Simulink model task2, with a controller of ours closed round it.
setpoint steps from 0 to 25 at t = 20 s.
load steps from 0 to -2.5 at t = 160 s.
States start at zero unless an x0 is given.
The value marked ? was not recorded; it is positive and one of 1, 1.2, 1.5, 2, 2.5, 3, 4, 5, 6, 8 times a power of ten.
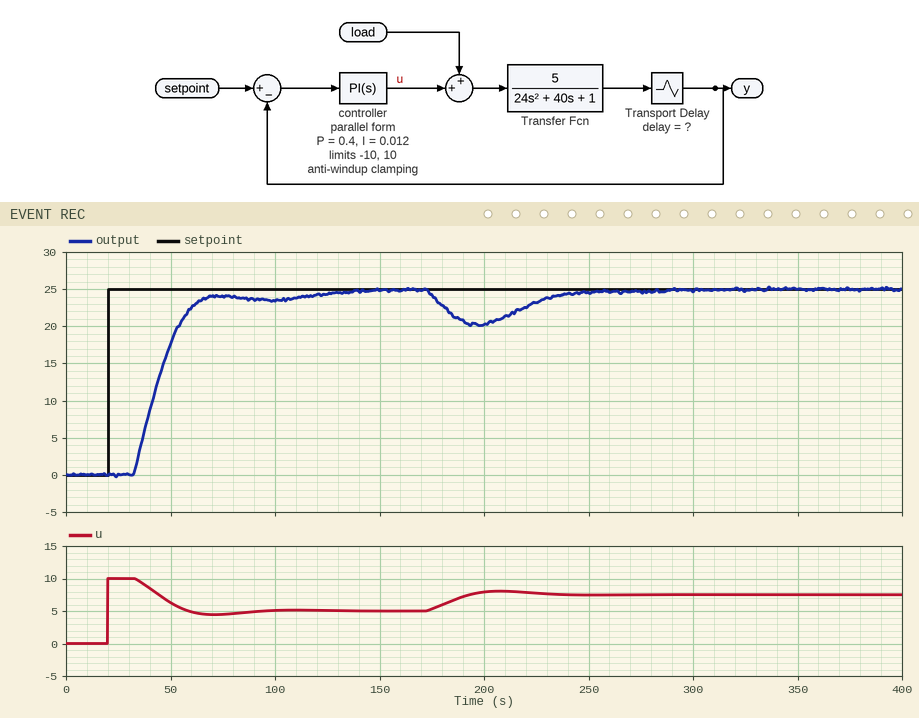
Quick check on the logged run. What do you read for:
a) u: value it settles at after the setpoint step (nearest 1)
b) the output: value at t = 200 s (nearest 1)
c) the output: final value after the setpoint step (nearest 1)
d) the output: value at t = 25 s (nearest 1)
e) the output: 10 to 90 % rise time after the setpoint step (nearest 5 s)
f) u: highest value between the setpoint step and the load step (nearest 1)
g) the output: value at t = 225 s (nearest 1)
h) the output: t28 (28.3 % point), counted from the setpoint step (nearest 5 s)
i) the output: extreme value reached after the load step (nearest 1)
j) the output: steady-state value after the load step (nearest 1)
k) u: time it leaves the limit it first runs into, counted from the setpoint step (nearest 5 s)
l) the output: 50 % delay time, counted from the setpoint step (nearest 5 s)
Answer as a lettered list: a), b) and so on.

a) 5
b) 20
c) 25
d) 0
e) 25 s
f) 10
g) 23
h) 20 s
i) 20
j) 25
k) 15 s
l) 25 s
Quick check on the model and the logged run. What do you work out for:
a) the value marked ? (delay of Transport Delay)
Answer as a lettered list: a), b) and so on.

a) 12
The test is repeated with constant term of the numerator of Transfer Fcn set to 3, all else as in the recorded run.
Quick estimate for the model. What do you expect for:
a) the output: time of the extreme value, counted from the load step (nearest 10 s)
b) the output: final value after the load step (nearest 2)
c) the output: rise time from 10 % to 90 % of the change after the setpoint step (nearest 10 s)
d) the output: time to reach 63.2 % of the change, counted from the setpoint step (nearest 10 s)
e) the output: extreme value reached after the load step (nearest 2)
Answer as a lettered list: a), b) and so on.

a) 40 s
b) 22
c) 60 s
d) 40 s
e) 22
